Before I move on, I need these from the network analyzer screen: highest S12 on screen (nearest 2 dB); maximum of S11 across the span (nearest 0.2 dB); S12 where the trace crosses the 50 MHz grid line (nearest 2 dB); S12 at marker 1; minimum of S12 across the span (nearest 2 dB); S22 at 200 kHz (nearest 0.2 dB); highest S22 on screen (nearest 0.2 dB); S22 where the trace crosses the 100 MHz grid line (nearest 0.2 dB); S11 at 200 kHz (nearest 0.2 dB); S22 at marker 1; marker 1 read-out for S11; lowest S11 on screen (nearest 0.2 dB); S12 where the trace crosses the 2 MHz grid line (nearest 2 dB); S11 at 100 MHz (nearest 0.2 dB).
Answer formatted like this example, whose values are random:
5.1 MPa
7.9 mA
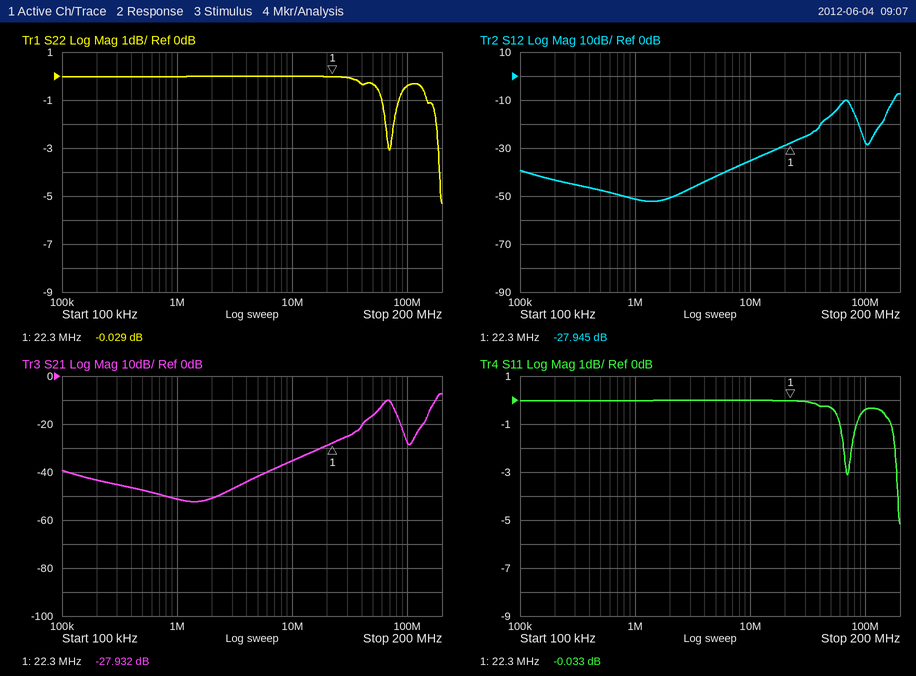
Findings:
-8 dB
0.0 dB
-16 dB
-27.945 dB
-52 dB
0.0 dB
0.0 dB
-0.4 dB
0.0 dB
-0.029 dB
-0.033 dB
-5.2 dB
-50 dB
-0.4 dB
